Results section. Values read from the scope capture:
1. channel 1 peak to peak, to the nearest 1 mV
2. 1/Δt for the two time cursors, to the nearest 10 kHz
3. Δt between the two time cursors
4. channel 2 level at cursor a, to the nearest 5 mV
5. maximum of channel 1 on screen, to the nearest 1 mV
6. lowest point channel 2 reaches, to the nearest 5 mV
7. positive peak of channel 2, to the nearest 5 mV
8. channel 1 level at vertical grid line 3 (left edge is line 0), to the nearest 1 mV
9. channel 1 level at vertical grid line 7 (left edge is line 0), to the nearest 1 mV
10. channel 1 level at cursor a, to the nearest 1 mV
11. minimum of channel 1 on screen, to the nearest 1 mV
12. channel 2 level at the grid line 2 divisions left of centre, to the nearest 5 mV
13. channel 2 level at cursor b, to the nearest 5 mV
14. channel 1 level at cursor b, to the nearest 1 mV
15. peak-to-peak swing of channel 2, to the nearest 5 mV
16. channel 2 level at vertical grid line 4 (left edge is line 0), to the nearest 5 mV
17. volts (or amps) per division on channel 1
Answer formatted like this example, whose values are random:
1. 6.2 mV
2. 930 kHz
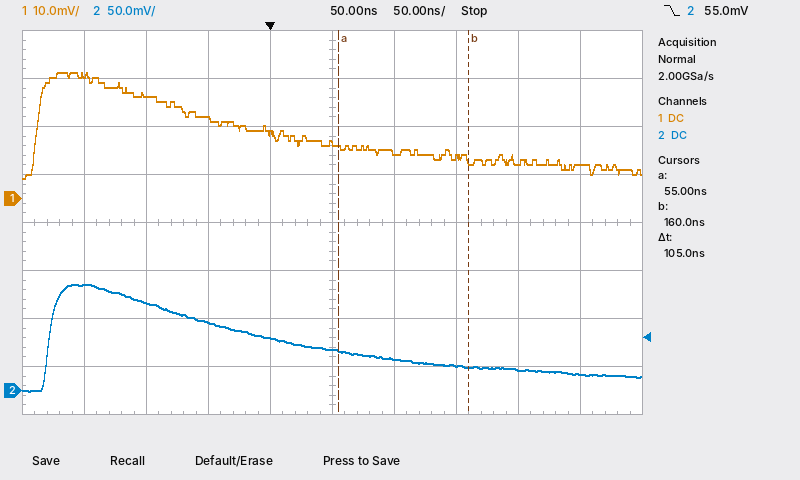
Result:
1. 22 mV
2. 9.52 MHz
3. 105 ns
4. 40 mV
5. 26 mV
6. 0 mV
7. 110 mV
8. 17 mV
9. 9 mV
10. 11 mV
11. 4 mV
12. 70 mV
13. 25 mV
14. 8 mV
15. 110 mV
16. 55 mV
17. 10 mV
